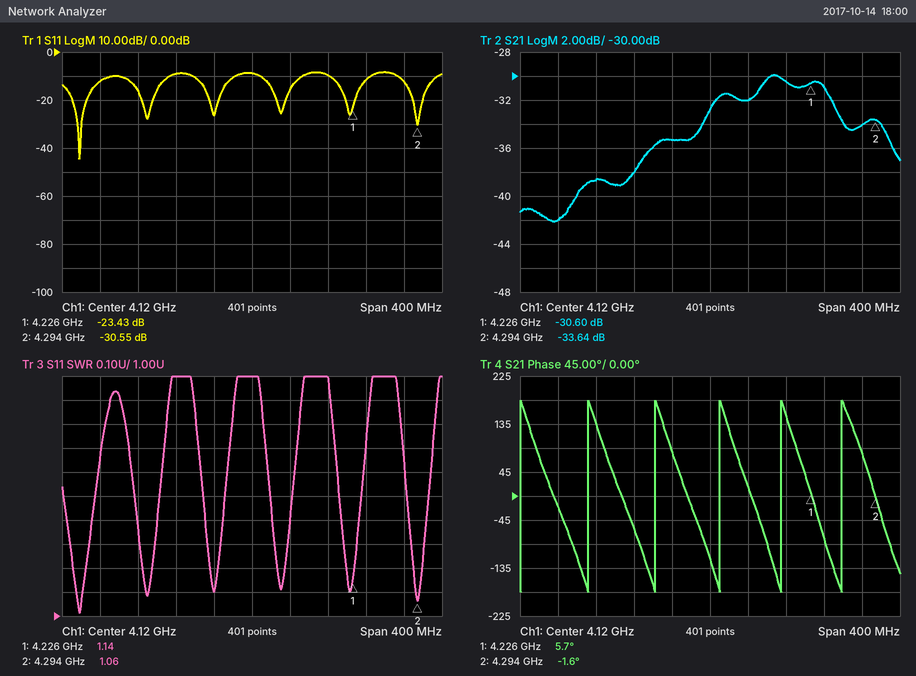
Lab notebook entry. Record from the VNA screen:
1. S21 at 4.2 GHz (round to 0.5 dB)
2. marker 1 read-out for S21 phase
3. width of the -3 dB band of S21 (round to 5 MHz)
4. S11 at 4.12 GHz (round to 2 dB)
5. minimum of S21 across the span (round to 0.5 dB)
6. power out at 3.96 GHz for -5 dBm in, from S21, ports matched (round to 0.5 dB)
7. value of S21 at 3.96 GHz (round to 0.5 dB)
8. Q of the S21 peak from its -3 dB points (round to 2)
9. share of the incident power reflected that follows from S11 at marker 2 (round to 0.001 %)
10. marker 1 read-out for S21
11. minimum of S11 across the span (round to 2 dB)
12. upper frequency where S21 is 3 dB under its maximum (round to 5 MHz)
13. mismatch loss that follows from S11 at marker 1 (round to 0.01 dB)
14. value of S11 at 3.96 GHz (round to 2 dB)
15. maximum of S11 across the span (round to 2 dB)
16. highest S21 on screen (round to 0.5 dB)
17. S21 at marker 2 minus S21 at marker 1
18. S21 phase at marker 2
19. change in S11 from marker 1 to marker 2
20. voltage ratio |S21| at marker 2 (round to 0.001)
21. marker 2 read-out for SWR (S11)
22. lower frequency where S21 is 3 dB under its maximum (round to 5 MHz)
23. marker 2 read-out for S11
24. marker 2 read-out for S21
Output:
-30.5 dB
5.7°
135 MHz
-8 dB
-42.0 dB
-47.0 dBm
-42.0 dB
32
0.088 %
-30.60 dB
-44 dB
4.255 GHz
0.02 dB
-12 dB
-8 dB
-30.0 dB
-3.04 dB
-1.6°
-7.12 dB
0.021
1.06
4.120 GHz
-30.55 dB
-33.64 dB
